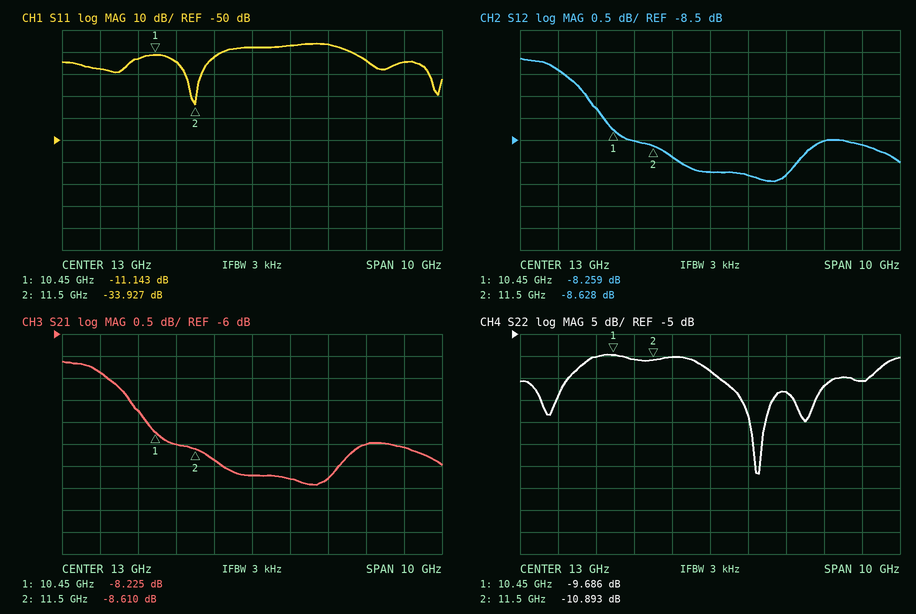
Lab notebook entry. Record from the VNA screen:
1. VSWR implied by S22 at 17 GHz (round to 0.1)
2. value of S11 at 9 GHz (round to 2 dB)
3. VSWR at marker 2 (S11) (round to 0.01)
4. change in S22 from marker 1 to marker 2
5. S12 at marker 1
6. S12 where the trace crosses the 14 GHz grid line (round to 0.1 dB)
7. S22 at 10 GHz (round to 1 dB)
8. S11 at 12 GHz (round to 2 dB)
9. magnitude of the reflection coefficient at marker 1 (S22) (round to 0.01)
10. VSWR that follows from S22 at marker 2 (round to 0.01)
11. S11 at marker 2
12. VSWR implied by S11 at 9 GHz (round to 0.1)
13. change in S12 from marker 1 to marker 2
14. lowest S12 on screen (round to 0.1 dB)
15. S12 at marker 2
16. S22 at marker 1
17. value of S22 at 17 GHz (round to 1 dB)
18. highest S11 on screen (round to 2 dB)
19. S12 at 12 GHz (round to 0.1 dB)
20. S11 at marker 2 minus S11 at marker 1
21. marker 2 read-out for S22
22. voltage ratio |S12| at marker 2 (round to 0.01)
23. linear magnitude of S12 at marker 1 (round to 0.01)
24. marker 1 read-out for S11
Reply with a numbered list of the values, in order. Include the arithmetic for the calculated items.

1. |Γ| = 10^(-16/20) = 0.1585; VSWR = (1 + 0.1585)/(1 − 0.1585) ≈ 1.4
2. -18 dB
3. (1 + 0.0201)/(1 − 0.0201) ≈ 1.04
4. -10.893 − (-9.686) = -1.207 dB
5. -8.259 dB
6. -9.3 dB
7. -10 dB
8. -12 dB
9. 10^(-9.686/20) ≈ 0.33
10. (1 + 0.2853)/(1 − 0.2853) ≈ 1.80
11. -33.927 dB
12. |Γ| = 10^(-18/20) = 0.1259; VSWR = (1 + 0.1259)/(1 − 0.1259) ≈ 1.3
13. -8.628 − (-8.259) = -0.369 dB
14. -9.4 dB
15. -8.628 dB
16. -9.686 dB
17. -16 dB
18. -6 dB
19. -8.9 dB
20. -33.927 − (-11.143) = -22.784 dB
21. -10.893 dB
22. 10^(-8.628/20) ≈ 0.37
23. 10^(-8.259/20) ≈ 0.39
24. -11.143 dB
